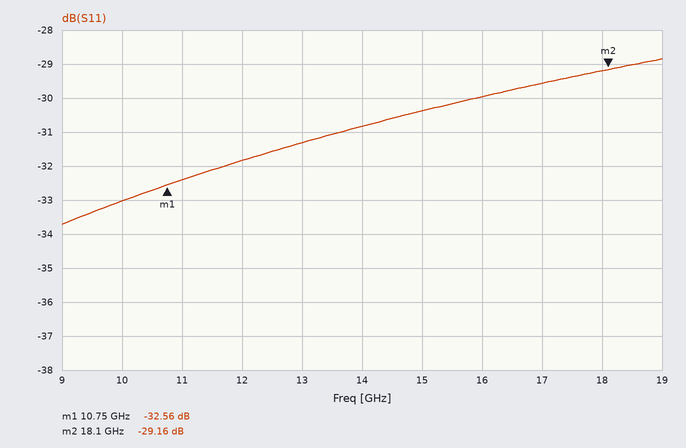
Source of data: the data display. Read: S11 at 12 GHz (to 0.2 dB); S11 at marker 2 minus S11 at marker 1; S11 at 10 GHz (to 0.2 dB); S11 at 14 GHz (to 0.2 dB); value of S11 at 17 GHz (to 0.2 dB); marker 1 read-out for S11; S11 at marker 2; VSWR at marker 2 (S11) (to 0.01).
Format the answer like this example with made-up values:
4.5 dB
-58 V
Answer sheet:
-31.8 dB
3.40 dB
-33.0 dB
-30.8 dB
-29.6 dB
-32.56 dB
-29.16 dB
1.07
